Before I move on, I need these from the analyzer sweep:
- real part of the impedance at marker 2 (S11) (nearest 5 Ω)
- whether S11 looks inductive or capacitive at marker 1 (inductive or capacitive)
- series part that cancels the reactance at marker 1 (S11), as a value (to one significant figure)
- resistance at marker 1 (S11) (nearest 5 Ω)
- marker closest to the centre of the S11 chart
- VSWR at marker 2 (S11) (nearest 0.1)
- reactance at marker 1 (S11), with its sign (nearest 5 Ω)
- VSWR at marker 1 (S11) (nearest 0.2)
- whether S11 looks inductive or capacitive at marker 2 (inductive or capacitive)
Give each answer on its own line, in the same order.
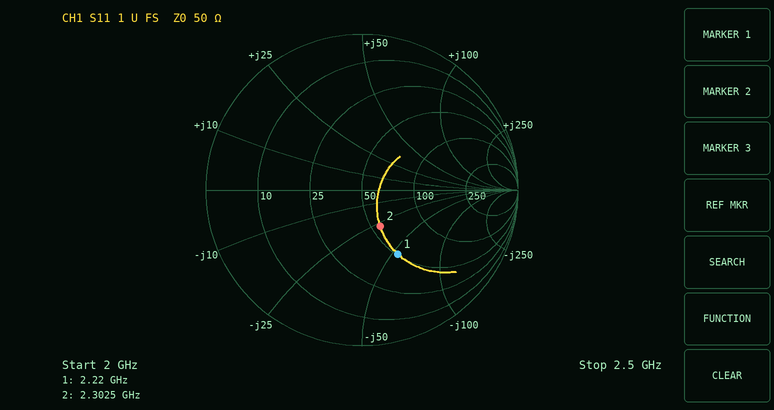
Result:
55 Ω
capacitive
4 nH
50 Ω
marker 2
1.7
-55 Ω
2.8
capacitive
